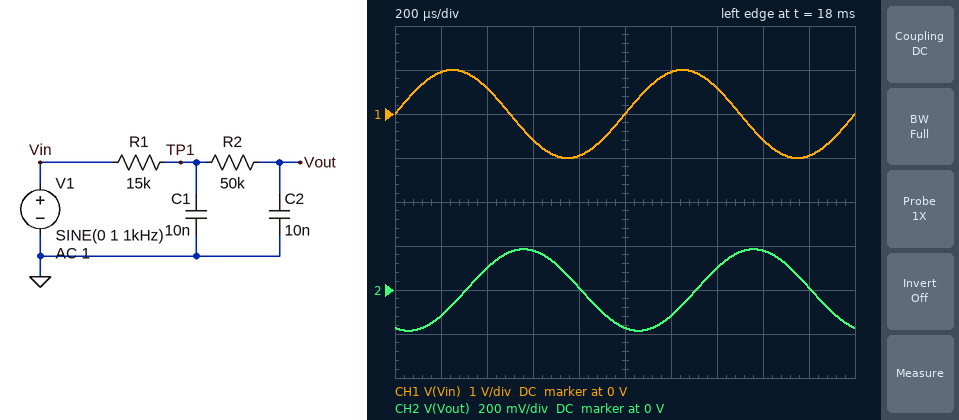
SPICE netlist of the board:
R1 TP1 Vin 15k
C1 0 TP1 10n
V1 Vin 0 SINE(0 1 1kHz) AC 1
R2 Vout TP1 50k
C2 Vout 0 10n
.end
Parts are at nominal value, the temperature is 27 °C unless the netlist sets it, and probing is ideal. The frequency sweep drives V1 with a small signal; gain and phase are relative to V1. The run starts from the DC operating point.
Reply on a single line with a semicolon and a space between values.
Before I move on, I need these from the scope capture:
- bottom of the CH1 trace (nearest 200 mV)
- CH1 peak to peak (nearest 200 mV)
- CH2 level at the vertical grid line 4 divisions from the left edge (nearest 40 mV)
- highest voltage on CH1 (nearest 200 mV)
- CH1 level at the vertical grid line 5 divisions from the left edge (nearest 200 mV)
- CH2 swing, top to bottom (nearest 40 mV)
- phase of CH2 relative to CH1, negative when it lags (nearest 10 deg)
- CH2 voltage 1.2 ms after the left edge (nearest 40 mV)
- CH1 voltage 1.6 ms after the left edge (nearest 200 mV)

-1.0 V; 2.0 V; 0 V; 1.0 V; 0 V; 360 mV; -110 deg; -120 mV; -600 mV
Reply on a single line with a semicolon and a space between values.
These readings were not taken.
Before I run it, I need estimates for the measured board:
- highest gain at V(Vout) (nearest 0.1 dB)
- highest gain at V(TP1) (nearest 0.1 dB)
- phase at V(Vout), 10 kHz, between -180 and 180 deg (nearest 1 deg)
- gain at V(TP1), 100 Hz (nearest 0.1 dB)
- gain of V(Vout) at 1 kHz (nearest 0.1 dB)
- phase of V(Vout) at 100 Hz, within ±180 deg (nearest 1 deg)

0 dB; 0 dB; -170 deg; -0.4 dB; -14.6 dB; -27 deg
